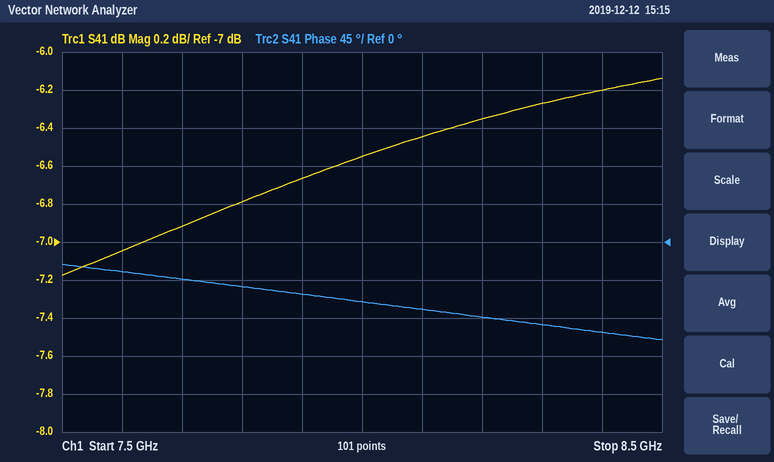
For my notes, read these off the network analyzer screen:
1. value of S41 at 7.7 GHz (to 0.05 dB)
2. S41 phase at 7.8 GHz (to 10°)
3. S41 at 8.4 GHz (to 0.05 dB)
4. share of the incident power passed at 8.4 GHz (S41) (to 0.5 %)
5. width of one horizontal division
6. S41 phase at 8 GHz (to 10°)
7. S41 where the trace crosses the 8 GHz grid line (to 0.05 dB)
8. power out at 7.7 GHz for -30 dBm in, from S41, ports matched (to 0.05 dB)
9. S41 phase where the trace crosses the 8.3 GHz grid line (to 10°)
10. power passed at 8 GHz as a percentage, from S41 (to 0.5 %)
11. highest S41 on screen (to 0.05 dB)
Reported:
-6.90 dB
-50°
-6.20 dB
24.0 %
100 MHz
-70°
-6.55 dB
-36.90 dBm
-100°
22.0 %
-6.15 dB
